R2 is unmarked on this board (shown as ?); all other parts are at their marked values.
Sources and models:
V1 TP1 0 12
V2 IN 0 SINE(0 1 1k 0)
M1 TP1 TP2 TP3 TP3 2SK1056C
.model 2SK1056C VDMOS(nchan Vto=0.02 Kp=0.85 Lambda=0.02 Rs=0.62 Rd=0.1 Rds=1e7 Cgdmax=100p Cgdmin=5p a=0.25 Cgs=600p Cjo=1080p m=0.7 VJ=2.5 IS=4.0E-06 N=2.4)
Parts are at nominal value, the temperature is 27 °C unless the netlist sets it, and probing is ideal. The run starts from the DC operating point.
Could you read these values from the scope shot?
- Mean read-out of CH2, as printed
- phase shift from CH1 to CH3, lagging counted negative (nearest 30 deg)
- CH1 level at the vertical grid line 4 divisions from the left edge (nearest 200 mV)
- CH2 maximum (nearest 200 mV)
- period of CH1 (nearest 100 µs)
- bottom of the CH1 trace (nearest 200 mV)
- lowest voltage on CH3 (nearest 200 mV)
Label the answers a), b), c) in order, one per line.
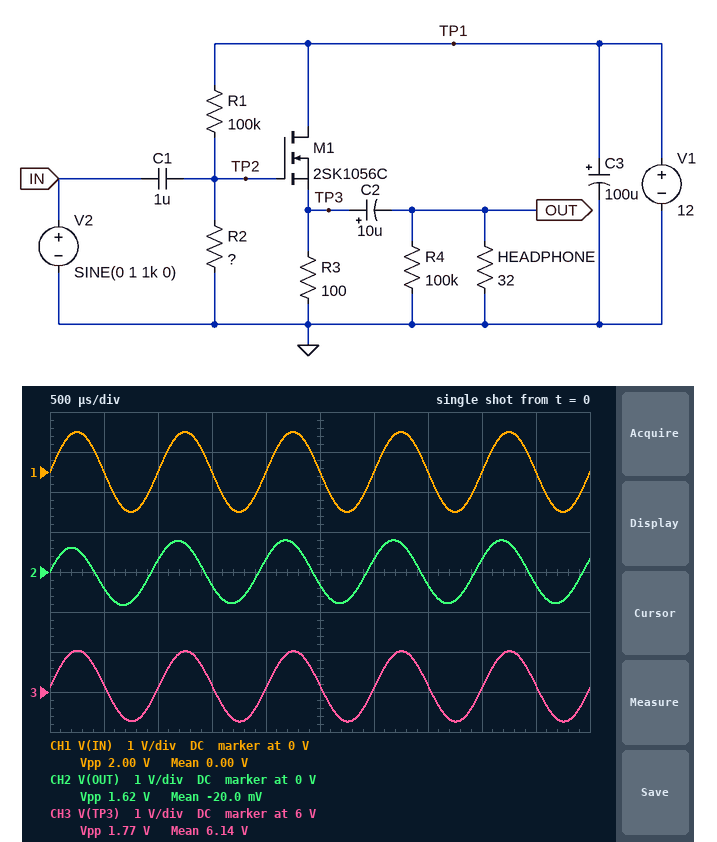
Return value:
a) -20.0 mV
b) 0 deg
c) 0 V
d) 800 mV
e) 1.0 ms
f) -1.0 V
g) 5.2 V
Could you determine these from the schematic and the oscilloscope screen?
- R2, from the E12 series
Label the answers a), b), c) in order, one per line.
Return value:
a) 120 kΩ
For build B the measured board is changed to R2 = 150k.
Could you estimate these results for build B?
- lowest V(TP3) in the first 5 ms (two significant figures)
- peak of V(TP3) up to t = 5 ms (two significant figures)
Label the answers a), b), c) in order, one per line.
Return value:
a) 5.9 V
b) 7.7 V
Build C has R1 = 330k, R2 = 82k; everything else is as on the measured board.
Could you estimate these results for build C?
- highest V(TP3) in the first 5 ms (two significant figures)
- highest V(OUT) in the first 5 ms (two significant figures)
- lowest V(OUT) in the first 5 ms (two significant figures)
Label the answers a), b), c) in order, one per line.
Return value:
a) 3.0 V
b) 710 mV
c) -580 mV
